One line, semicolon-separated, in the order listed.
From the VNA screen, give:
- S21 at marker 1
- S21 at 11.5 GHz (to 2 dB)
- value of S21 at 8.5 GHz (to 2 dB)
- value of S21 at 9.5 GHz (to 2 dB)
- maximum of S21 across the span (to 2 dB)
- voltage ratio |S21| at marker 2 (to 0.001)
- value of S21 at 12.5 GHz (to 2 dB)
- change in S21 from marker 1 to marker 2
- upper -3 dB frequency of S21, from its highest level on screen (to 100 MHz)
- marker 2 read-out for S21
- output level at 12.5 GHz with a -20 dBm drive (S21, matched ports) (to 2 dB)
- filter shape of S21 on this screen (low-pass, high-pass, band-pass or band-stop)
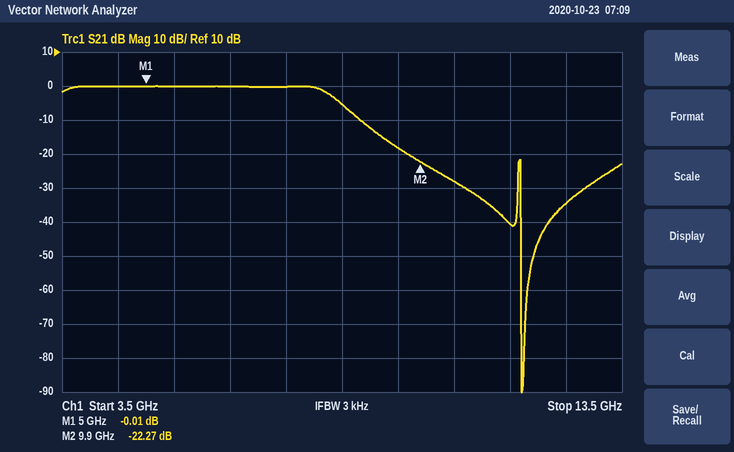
-0.01 dB; -40 dB; -6 dB; -18 dB; 0 dB; 0.077; -34 dB; -22.26 dB; 8.3 GHz; -22.27 dB; -54 dBm; low-pass
